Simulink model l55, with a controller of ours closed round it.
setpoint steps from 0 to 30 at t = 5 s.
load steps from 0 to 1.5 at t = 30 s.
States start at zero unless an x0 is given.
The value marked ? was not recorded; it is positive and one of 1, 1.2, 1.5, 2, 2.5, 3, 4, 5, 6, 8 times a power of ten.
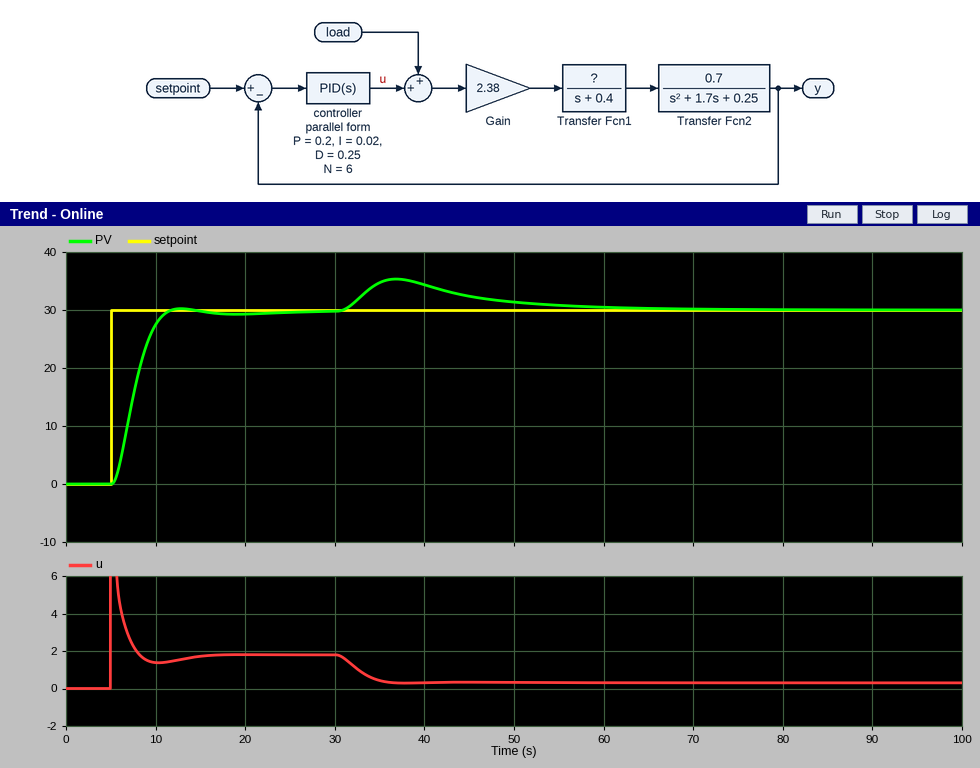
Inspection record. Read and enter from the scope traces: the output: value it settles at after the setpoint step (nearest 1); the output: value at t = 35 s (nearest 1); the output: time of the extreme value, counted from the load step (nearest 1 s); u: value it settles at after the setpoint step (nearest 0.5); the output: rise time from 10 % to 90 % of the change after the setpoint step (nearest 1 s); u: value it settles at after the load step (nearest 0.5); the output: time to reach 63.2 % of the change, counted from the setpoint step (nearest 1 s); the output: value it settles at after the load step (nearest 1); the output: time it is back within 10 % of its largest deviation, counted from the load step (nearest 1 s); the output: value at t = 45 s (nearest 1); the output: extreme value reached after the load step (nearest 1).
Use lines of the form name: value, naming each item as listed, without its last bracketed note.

the output: value it settles at after the setpoint step: 30
the output: value at t = 35 s: 35
the output: time of the extreme value, counted from the load step: 7 s
u: value it settles at after the setpoint step: 2.0
the output: rise time from 10 % to 90 % of the change after the setpoint step: 4 s
u: value it settles at after the load step: 0.5
the output: time to reach 63.2 % of the change, counted from the setpoint step: 3 s
the output: value it settles at after the load step: 30
the output: time it is back within 10 % of its largest deviation, counted from the load step: 28 s
the output: value at t = 45 s: 32
the output: extreme value reached after the load step: 35
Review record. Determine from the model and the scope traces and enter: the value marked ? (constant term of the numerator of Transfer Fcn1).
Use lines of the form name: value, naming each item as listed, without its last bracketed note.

the value marked ?: 1
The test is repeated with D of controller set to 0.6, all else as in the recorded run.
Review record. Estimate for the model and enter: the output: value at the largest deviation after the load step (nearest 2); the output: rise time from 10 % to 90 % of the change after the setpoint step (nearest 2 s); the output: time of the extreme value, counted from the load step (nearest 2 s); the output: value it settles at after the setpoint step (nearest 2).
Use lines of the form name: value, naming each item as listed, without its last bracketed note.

the output: value at the largest deviation after the load step: 34
the output: rise time from 10 % to 90 % of the change after the setpoint step: 8 s
the output: time of the extreme value, counted from the load step: 8 s
the output: value it settles at after the setpoint step: 30
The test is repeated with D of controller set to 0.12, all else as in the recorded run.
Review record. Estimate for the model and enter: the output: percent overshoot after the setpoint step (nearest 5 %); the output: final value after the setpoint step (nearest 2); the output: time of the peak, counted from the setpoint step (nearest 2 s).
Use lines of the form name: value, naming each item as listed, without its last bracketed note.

the output: percent overshoot after the setpoint step: 10 %
the output: final value after the setpoint step: 30
the output: time of the peak, counted from the setpoint step: 8 s
